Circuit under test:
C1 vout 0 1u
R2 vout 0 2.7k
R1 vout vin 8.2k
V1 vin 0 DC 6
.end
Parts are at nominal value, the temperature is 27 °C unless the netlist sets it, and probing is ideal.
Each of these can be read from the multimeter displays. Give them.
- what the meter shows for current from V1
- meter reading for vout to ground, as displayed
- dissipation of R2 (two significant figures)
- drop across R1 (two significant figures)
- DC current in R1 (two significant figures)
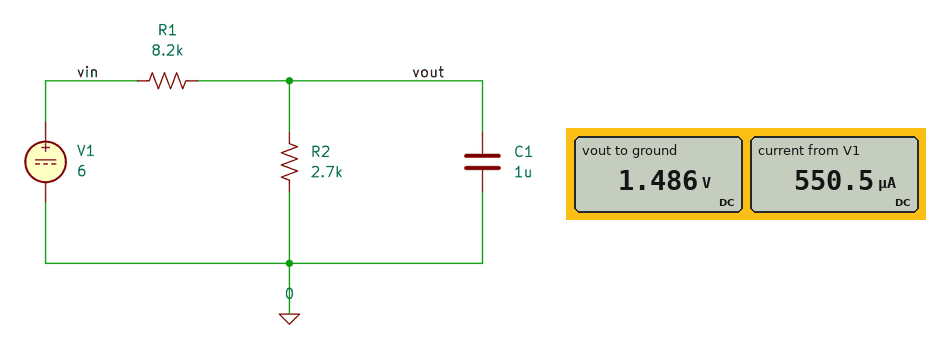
550.5 µA
1.486 V
820 µW
4.5 V
550 µA
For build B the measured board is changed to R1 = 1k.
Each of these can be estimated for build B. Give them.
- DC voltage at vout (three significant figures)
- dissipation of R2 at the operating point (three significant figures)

4.38 V
7.10 mW
